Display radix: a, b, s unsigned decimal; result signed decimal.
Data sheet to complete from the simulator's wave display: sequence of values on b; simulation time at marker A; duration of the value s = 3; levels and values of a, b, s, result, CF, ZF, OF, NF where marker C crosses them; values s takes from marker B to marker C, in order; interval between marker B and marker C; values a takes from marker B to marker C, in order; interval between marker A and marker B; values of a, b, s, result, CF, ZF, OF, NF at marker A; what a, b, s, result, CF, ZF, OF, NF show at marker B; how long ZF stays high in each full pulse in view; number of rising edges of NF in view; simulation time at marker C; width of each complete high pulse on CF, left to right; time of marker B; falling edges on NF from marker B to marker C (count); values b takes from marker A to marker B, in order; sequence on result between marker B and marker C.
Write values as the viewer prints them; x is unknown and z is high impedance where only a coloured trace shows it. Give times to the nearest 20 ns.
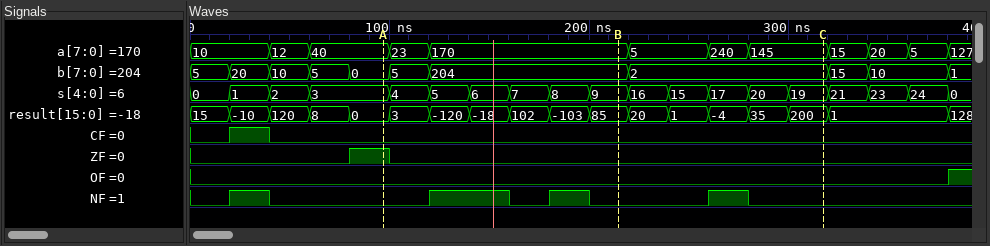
5, 20, 10, 5, 0, 5, 204, 2, 15, 10, 1
100 ns
40 ns
a=145, b=2, s=19, result=200, CF=0, ZF=0, OF=0, NF=0
9, 16, 15, 17, 20, 19
100 ns
170, 5, 240, 145
120 ns
a=40, b=0, s=3, result=0, CF=0, ZF=1, OF=0, NF=0
a=170, b=204, s=9, result=85, CF=0, ZF=0, OF=0, NF=0
20 ns
4
320 ns
20 ns
220 ns
1
0, 5, 204
85, 20, 1, -4, 35, 200
